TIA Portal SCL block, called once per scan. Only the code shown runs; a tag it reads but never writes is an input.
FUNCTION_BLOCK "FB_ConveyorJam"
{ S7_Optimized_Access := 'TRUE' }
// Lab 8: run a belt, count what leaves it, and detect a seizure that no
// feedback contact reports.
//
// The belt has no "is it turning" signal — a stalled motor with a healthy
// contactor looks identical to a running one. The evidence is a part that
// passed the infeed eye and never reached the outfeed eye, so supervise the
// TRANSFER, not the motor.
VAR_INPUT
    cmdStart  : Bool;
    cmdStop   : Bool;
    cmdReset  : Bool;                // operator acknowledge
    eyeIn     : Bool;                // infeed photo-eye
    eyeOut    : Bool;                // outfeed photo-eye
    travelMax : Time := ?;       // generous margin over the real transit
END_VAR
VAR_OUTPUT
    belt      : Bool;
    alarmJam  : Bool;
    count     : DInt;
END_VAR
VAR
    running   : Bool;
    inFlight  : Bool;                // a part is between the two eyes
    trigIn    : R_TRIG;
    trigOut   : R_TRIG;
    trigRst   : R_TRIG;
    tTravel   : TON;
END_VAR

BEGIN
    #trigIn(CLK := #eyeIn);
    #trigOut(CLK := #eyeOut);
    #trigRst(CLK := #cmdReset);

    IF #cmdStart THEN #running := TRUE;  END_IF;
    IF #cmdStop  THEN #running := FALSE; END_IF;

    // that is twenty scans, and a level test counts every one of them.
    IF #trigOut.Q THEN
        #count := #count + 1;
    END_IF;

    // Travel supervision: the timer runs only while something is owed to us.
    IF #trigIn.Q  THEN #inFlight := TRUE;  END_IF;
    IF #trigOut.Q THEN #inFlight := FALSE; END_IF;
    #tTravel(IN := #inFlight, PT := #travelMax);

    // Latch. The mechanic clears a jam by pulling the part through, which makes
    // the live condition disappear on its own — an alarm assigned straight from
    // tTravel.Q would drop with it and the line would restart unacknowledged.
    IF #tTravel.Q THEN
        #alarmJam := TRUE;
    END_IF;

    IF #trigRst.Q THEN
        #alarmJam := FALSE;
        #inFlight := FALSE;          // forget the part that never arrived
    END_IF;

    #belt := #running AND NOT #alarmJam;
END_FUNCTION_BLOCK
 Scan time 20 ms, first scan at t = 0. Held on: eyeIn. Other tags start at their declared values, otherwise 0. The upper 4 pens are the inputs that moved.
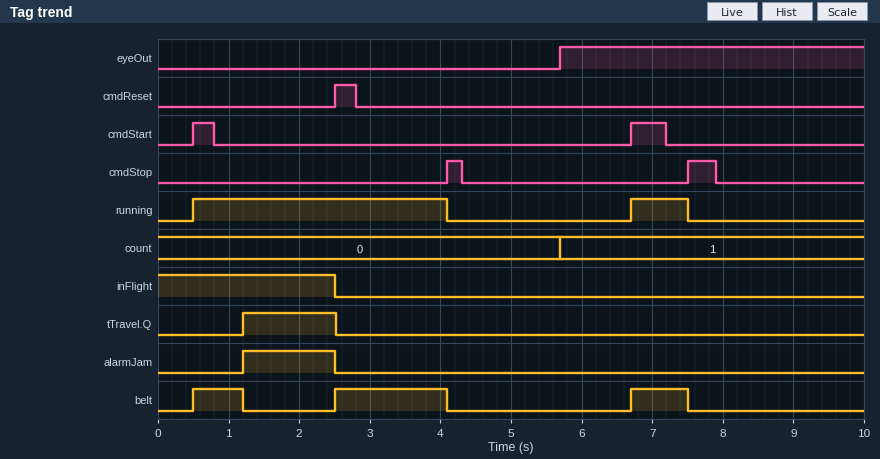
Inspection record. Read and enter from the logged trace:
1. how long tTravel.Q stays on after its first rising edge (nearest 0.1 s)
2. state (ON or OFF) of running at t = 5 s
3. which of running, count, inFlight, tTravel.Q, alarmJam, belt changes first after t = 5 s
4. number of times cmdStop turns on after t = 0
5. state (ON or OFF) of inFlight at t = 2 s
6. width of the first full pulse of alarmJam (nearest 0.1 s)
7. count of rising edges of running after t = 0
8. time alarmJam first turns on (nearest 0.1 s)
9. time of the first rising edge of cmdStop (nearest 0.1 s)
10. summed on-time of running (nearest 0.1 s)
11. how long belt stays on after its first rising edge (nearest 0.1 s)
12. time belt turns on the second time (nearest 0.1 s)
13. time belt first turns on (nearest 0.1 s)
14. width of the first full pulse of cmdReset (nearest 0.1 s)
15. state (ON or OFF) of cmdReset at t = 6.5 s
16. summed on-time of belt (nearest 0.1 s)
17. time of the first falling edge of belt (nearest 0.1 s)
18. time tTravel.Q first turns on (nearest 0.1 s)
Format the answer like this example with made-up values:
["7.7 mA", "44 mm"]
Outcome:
["1.3 s", "OFF", "count", "2", "ON", "1.3 s", "2", "1.2 s", "4.1 s", "4.4 s", "0.7 s", "2.5 s", "0.5 s", "0.3 s", "OFF", "3.1 s", "1.2 s", "1.2 s"]
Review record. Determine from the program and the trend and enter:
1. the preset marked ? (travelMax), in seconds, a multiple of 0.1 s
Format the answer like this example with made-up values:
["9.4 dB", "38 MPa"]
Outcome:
["1.2 s"]
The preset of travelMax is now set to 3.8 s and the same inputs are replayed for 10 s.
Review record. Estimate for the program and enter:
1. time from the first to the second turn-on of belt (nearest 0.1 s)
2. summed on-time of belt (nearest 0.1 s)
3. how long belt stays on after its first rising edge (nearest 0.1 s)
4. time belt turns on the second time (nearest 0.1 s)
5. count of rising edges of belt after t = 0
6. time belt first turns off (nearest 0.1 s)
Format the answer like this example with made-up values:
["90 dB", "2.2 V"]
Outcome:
["6.2 s", "4.4 s", "3.6 s", "6.7 s", "2", "4.1 s"]
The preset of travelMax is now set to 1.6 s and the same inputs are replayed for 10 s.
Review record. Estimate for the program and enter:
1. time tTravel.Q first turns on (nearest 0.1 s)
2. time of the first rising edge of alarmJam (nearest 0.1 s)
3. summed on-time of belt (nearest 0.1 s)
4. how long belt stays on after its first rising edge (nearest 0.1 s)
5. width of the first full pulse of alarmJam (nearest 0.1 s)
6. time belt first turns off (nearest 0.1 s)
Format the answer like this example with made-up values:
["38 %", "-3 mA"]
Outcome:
["1.6 s", "1.6 s", "3.5 s", "1.1 s", "0.9 s", "1.6 s"]
